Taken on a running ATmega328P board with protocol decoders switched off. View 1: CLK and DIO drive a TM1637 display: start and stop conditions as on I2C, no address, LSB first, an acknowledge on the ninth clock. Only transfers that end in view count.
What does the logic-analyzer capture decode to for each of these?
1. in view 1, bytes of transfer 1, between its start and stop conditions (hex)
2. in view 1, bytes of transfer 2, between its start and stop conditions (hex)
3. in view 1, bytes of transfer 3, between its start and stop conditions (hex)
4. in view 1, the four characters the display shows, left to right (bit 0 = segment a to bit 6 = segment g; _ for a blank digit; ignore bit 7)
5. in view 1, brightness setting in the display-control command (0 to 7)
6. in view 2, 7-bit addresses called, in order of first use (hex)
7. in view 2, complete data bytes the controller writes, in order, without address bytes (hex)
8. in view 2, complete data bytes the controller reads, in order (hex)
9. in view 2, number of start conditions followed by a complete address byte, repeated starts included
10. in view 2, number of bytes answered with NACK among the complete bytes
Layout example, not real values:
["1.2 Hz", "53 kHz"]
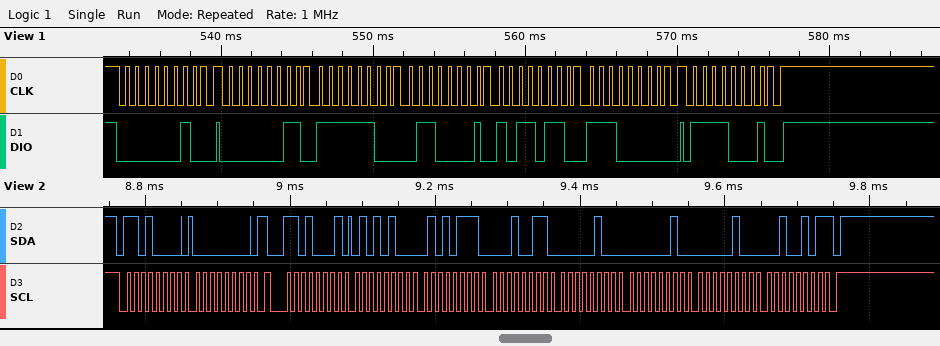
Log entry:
["40", "C0 3F 86 6D 07", "8F", "0157", "7", "0x68", "00", "54 57 13 04 02 04 25", "2", "1"]
